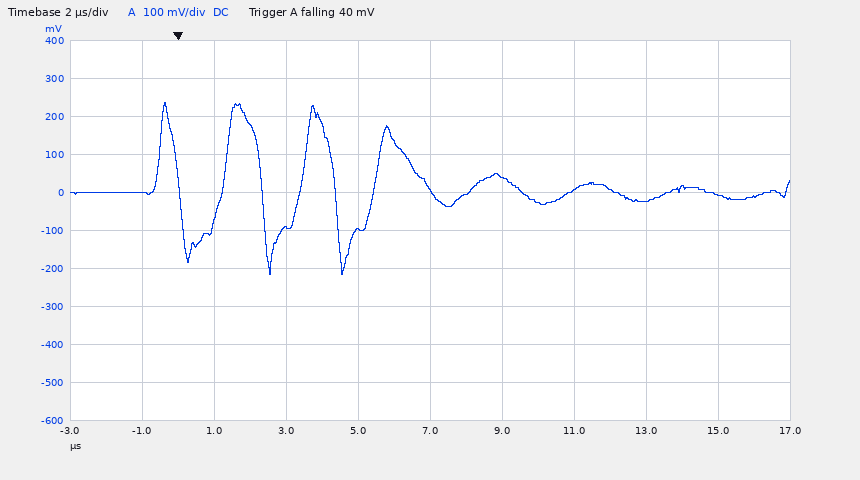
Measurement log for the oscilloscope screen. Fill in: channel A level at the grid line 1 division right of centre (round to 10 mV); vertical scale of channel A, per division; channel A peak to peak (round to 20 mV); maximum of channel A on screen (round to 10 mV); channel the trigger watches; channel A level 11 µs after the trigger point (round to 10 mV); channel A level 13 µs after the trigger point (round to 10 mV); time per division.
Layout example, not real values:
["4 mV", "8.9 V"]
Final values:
["40 mV", "100 mV", "460 mV", "240 mV", "channel A", "10 mV", "-20 mV", "2 µs"]
